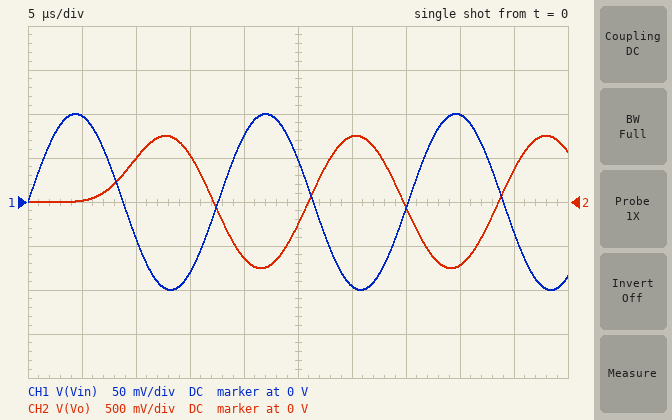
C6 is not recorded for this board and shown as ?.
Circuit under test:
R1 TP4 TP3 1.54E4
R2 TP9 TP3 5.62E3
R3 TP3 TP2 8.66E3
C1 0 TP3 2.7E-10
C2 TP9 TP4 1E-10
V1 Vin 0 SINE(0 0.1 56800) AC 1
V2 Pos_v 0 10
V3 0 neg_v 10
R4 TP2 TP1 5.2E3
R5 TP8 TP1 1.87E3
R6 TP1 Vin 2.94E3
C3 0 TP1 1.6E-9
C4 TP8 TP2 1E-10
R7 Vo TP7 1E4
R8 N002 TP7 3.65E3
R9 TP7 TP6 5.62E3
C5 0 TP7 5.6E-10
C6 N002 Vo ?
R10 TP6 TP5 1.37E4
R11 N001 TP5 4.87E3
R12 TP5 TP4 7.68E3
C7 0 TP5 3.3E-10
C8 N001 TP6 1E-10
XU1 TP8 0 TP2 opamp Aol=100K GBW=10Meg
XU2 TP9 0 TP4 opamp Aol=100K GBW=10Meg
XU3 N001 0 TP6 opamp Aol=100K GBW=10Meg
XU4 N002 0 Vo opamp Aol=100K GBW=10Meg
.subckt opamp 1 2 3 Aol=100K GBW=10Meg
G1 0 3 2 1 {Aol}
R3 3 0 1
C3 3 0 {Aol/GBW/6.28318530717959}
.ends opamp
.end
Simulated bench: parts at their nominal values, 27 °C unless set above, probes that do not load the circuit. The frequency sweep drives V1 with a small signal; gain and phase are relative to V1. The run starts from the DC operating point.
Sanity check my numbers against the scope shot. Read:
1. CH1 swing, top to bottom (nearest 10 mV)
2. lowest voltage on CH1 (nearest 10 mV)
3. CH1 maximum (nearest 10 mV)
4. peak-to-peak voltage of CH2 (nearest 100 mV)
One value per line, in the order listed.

200 mV
-100 mV
100 mV
1.5 V
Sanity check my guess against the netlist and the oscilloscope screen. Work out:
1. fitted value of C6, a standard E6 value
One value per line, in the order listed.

68 pF
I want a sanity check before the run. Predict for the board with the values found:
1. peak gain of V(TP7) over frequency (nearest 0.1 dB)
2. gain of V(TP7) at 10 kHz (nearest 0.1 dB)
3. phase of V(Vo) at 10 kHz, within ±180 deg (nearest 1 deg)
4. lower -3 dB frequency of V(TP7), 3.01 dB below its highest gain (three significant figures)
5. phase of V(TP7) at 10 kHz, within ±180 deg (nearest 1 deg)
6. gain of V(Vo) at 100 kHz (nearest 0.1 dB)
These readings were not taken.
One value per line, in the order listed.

-2.3 dB
-15.7 dB
-30 deg
37.0 kHz
-120 deg
12.1 dB
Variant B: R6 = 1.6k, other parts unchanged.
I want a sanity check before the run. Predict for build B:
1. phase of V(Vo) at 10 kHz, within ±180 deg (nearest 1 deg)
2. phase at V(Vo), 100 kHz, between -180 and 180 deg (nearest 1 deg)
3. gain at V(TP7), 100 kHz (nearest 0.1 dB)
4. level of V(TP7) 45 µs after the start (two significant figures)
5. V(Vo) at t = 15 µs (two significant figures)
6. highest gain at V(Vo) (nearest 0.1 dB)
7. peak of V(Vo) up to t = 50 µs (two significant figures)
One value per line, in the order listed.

-31 deg
49 deg
0 dB
-110 mV
1.0 V
25.3 dB
1.3 V
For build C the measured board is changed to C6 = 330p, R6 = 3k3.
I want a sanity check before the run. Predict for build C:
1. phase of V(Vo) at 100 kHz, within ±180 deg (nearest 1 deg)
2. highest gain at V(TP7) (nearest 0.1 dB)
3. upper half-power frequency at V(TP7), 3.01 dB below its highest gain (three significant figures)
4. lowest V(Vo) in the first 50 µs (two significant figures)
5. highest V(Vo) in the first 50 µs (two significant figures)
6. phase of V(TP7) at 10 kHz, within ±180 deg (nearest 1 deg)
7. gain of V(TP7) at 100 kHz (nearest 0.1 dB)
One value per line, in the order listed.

8 deg
2.3 dB
76.7 kHz
-270 mV
380 mV
-138 deg
-4.3 dB
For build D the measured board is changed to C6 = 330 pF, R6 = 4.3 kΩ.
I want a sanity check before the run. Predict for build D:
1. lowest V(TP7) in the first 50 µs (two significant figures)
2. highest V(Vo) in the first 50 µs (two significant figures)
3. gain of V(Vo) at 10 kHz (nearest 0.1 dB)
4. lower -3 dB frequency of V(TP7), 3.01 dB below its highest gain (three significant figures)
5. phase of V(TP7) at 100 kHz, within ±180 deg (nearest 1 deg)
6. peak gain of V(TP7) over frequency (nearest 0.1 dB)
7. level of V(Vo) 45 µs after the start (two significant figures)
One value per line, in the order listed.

-91 mV
300 mV
16.1 dB
16.0 kHz
-80 deg
0 dB
-84 mV
